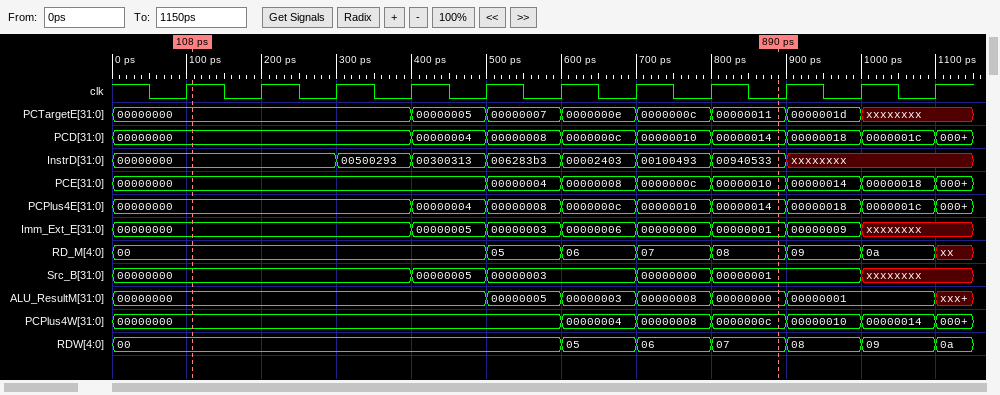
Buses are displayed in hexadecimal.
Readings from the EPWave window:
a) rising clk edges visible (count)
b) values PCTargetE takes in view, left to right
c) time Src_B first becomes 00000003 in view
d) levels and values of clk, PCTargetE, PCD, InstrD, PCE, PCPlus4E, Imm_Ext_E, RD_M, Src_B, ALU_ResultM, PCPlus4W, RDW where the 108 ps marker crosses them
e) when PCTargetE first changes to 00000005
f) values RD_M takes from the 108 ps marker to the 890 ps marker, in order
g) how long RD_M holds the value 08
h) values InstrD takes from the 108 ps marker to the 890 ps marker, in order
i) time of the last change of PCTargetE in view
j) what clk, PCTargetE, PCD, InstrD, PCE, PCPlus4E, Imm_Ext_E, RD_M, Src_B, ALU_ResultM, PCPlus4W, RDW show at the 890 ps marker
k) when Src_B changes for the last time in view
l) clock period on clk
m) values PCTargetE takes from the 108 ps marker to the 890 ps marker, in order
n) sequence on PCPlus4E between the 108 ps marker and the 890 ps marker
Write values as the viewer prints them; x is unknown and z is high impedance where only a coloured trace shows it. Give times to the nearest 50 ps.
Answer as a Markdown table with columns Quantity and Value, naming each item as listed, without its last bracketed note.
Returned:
| Quantity | Value |
|---|---|
| rising clk edges visible | 11 |
| values PCTargetE takes in view, left to right | 00000000, 00000005, 00000007, 0000000e, 0000000c, 00000011, 0000001d, xxxxxxxx |
| time Src_B first becomes 00000003 in view | 500 ps |
| levels and values of clk, PCTargetE, PCD, InstrD, PCE, PCPlus4E, Imm_Ext_E, RD_M, Src_B, ALU_ResultM, PCPlus4W, RDW where the 108 ps marker crosses them | clk=1, PCTargetE=00000000, PCD=00000000, InstrD=00000000, PCE=00000000, PCPlus4E=00000000, Imm_Ext_E=00000000, RD_M=00, Src_B=00000000, ALU_ResultM=00000000, PCPlus4W=00000000, RDW=00 |
| when PCTargetE first changes to 00000005 | 400 ps |
| values RD_M takes from the 108 ps marker to the 890 ps marker, in order | 00, 05, 06, 07, 08 |
| how long RD_M holds the value 08 | 100 ps |
| values InstrD takes from the 108 ps marker to the 890 ps marker, in order | 00000000, 00500293, 00300313, 006283b3, 00002403, 00100493, 00940533 |
| time of the last change of PCTargetE in view | 1000 ps |
| what clk, PCTargetE, PCD, InstrD, PCE, PCPlus4E, Imm_Ext_E, RD_M, Src_B, ALU_ResultM, PCPlus4W, RDW show at the 890 ps marker | clk=0, PCTargetE=00000011, PCD=00000014, InstrD=00940533, PCE=00000010, PCPlus4E=00000014, Imm_Ext_E=00000001, RD_M=08, Src_B=00000001, ALU_ResultM=00000000, PCPlus4W=0000000c, RDW=07 |
| when Src_B changes for the last time in view | 1000 ps |
| clock period on clk | 100 ps |
| values PCTargetE takes from the 108 ps marker to the 890 ps marker, in order | 00000000, 00000005, 00000007, 0000000e, 0000000c, 00000011 |
| sequence on PCPlus4E between the 108 ps marker and the 890 ps marker | 00000000, 00000004, 00000008, 0000000c, 00000010, 00000014 |
